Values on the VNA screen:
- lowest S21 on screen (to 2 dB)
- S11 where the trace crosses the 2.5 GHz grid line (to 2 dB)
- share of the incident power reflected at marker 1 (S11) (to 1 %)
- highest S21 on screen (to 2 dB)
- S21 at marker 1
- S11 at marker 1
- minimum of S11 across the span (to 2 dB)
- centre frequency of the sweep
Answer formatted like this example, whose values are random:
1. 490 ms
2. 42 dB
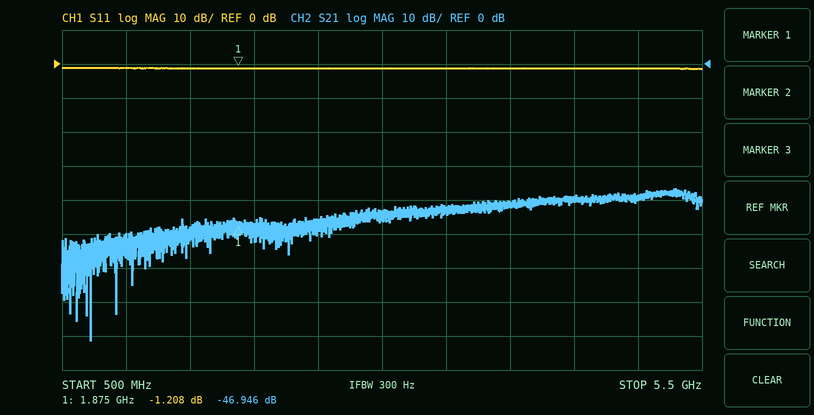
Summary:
1. -82 dB
2. -2 dB
3. 76 %
4. -36 dB
5. -46.946 dB
6. -1.208 dB
7. -2 dB
8. 3 GHz
